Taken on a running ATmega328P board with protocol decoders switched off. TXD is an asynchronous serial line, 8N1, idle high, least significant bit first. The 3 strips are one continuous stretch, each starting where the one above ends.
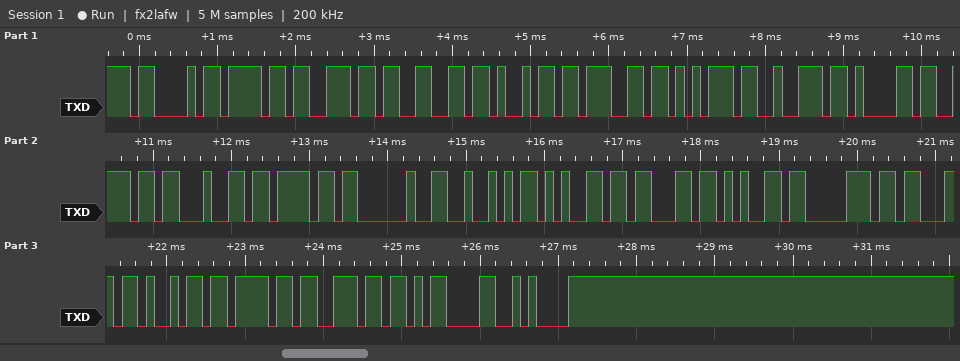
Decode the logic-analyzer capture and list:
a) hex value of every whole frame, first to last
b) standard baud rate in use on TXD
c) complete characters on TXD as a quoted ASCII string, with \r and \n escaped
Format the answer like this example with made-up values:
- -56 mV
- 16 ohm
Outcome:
- 43 6F 6E 66 69 67 75 72 61 6E 64 6F 20 52 65 63 65 70 63 69 6F 6E 0D 0A
- 9600 baud
- "Configurando Recepcion\r\n"
